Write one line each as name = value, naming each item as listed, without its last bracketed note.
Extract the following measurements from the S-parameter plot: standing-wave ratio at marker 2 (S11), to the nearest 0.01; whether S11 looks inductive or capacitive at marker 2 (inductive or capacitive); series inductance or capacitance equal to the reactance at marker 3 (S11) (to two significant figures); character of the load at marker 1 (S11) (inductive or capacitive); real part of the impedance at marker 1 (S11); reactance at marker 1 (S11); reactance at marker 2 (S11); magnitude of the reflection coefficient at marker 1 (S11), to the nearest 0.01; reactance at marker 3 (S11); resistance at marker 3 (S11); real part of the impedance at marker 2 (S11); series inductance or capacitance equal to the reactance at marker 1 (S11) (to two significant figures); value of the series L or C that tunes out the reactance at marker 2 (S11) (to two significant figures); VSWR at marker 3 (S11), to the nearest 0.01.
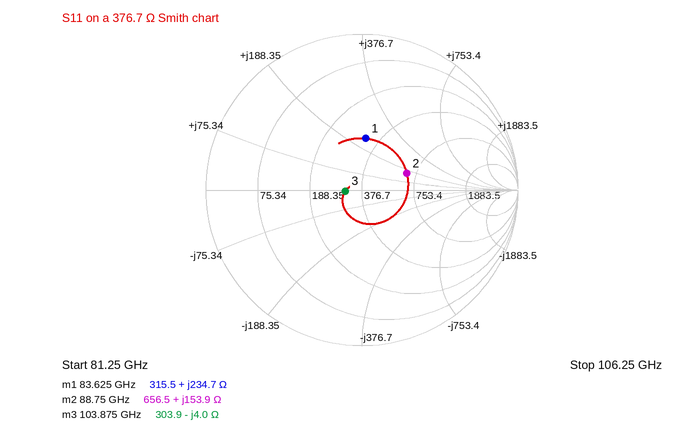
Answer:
standing-wave ratio at marker 2 (S11), to the nearest 0.01 = 1.88
whether S11 looks inductive or capacitive at marker 2 = inductive
series inductance or capacitance equal to the reactance at marker 3 (S11) = 380 fF
character of the load at marker 1 (S11) = inductive
real part of the impedance at marker 1 = 315.5 Ω
reactance at marker 1 = +234.7 Ω
reactance at marker 2 = +153.9 Ω
magnitude of the reflection coefficient at marker 1 (S11), to the nearest 0.01 = 0.33
reactance at marker 3 = -4.0 Ω
resistance at marker 3 = 303.9 Ω
real part of the impedance at marker 2 = 656.5 Ω
series inductance or capacitance equal to the reactance at marker 1 (S11) = 450 pH
value of the series L or C that tunes out the reactance at marker 2 (S11) = 12 fF
VSWR at marker 3 (S11), to the nearest 0.01 = 1.24
